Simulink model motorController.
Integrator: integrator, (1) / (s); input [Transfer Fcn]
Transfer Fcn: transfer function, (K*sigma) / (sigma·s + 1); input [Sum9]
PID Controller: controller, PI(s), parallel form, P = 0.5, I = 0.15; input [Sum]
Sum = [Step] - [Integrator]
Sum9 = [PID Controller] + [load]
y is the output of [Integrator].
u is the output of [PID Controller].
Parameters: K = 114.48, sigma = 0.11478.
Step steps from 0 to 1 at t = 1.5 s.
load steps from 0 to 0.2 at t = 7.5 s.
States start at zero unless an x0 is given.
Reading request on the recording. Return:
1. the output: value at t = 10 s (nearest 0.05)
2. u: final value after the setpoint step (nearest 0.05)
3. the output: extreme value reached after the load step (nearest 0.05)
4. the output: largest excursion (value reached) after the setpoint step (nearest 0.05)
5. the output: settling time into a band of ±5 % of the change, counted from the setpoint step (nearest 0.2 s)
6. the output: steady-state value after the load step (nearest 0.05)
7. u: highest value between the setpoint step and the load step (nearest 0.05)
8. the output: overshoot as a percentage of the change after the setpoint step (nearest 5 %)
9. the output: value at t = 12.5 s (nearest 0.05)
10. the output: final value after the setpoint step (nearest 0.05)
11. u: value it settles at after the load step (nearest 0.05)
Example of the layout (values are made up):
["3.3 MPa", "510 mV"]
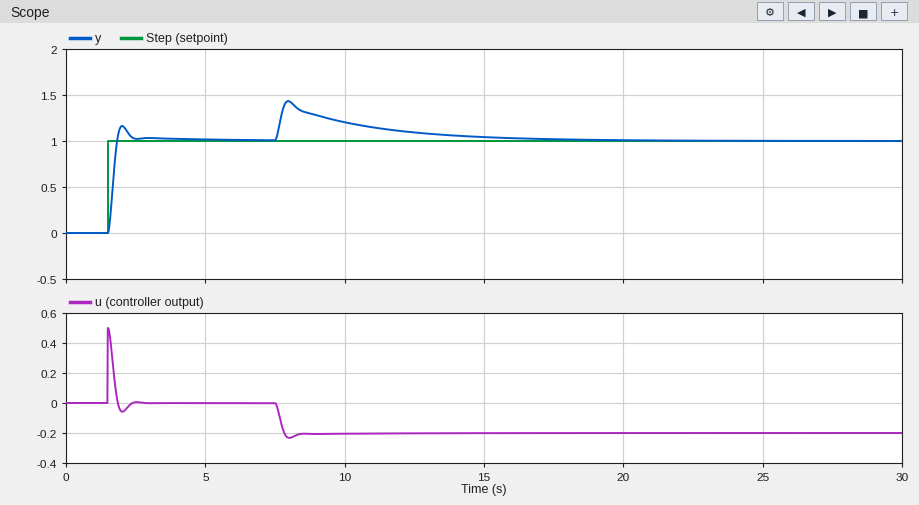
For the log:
["1.20", "0.00", "1.45", "1.15", "0.8 s", "1.00", "0.50", "15 %", "1.10", "1.00", "-0.20"]
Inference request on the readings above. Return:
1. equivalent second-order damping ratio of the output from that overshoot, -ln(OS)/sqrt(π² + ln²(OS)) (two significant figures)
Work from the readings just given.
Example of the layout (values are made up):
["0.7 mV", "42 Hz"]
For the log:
["0.52"]
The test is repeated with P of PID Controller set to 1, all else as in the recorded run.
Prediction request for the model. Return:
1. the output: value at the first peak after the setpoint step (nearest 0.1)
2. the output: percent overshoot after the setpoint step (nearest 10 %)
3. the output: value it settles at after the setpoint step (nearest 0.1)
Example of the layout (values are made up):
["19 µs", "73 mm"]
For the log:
["1.3", "30 %", "1.0"]
